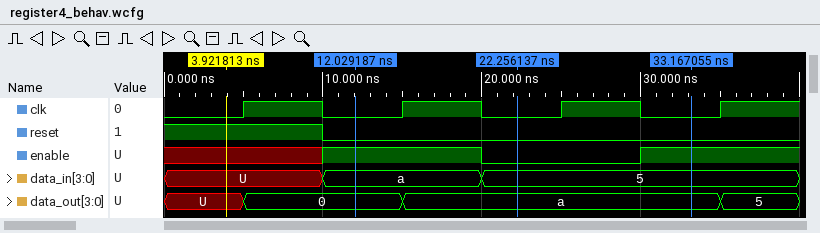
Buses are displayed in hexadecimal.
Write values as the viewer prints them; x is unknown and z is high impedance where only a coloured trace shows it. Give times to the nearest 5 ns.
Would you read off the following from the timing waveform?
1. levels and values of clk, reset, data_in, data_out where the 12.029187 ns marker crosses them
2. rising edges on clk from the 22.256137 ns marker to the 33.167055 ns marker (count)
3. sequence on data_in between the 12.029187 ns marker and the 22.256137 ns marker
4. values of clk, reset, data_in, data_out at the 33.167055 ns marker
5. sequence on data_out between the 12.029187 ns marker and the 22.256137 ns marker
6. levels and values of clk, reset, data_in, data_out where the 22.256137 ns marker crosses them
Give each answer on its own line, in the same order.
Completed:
clk=0, reset=0, data_in=a, data_out=0
1
a, 5
clk=0, reset=0, data_in=5, data_out=a
0, a
clk=0, reset=0, data_in=5, data_out=a
